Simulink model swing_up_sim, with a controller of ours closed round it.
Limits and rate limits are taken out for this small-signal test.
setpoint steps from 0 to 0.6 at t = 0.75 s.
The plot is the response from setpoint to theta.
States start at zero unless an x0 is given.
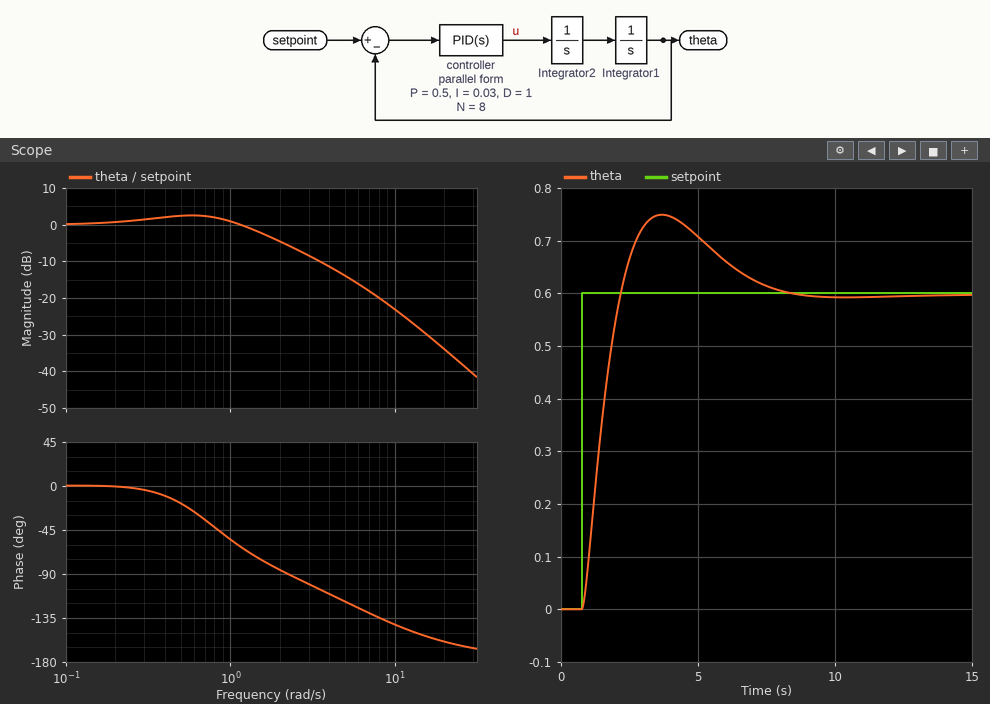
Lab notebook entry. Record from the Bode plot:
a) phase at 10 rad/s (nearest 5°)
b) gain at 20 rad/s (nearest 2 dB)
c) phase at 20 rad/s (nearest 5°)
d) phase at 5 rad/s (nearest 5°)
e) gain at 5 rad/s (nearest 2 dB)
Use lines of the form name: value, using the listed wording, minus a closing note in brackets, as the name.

phase at 10 rad/s: -140°
gain at 20 rad/s: -34 dB
phase at 20 rad/s: -160°
phase at 5 rad/s: -120°
gain at 5 rad/s: -14 dB
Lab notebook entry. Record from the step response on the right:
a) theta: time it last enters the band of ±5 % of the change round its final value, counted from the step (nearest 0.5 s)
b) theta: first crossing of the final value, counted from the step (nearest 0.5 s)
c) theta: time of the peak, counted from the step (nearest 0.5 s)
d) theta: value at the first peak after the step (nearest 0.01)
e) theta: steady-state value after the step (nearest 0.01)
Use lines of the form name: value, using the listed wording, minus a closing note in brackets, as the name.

theta: time it last enters the band of ±5 % of the change round its final value, counted from the step: 6.0 s
theta: first crossing of the final value, counted from the step: 1.5 s
theta: time of the peak, counted from the step: 3.0 s
theta: value at the first peak after the step: 0.75
theta: steady-state value after the step: 0.60
